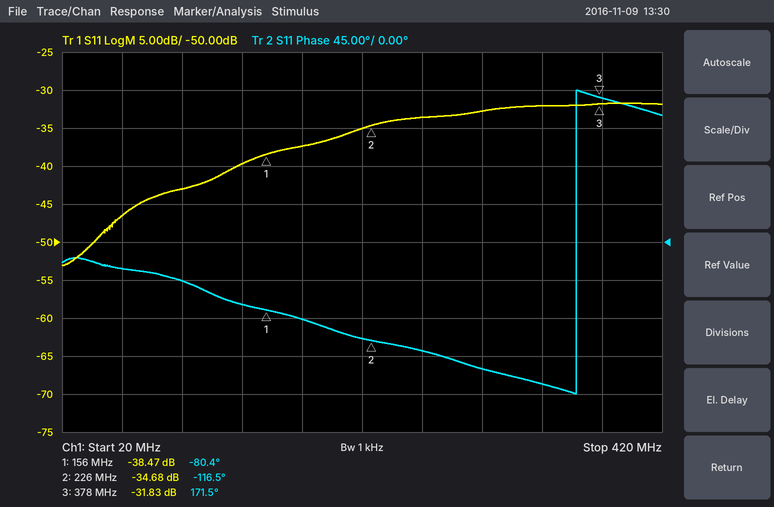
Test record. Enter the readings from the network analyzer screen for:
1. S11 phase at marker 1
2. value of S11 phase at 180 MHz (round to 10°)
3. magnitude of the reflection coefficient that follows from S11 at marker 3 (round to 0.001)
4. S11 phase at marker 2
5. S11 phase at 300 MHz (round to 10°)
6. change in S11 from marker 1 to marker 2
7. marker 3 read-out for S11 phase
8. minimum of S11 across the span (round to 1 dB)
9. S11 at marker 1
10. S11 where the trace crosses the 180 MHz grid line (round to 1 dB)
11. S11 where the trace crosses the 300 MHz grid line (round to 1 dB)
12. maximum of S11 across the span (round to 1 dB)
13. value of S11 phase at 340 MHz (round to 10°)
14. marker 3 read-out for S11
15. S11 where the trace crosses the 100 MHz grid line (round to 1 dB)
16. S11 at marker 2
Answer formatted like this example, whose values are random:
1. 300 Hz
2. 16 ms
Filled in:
1. -80.4°
2. -90°
3. 0.026
4. -116.5°
5. -150°
6. 3.79 dB
7. 171.5°
8. -53 dB
9. -38.47 dB
10. -37 dB
11. -33 dB
12. -32 dB
13. -170°
14. -31.83 dB
15. -43 dB
16. -34.68 dB
